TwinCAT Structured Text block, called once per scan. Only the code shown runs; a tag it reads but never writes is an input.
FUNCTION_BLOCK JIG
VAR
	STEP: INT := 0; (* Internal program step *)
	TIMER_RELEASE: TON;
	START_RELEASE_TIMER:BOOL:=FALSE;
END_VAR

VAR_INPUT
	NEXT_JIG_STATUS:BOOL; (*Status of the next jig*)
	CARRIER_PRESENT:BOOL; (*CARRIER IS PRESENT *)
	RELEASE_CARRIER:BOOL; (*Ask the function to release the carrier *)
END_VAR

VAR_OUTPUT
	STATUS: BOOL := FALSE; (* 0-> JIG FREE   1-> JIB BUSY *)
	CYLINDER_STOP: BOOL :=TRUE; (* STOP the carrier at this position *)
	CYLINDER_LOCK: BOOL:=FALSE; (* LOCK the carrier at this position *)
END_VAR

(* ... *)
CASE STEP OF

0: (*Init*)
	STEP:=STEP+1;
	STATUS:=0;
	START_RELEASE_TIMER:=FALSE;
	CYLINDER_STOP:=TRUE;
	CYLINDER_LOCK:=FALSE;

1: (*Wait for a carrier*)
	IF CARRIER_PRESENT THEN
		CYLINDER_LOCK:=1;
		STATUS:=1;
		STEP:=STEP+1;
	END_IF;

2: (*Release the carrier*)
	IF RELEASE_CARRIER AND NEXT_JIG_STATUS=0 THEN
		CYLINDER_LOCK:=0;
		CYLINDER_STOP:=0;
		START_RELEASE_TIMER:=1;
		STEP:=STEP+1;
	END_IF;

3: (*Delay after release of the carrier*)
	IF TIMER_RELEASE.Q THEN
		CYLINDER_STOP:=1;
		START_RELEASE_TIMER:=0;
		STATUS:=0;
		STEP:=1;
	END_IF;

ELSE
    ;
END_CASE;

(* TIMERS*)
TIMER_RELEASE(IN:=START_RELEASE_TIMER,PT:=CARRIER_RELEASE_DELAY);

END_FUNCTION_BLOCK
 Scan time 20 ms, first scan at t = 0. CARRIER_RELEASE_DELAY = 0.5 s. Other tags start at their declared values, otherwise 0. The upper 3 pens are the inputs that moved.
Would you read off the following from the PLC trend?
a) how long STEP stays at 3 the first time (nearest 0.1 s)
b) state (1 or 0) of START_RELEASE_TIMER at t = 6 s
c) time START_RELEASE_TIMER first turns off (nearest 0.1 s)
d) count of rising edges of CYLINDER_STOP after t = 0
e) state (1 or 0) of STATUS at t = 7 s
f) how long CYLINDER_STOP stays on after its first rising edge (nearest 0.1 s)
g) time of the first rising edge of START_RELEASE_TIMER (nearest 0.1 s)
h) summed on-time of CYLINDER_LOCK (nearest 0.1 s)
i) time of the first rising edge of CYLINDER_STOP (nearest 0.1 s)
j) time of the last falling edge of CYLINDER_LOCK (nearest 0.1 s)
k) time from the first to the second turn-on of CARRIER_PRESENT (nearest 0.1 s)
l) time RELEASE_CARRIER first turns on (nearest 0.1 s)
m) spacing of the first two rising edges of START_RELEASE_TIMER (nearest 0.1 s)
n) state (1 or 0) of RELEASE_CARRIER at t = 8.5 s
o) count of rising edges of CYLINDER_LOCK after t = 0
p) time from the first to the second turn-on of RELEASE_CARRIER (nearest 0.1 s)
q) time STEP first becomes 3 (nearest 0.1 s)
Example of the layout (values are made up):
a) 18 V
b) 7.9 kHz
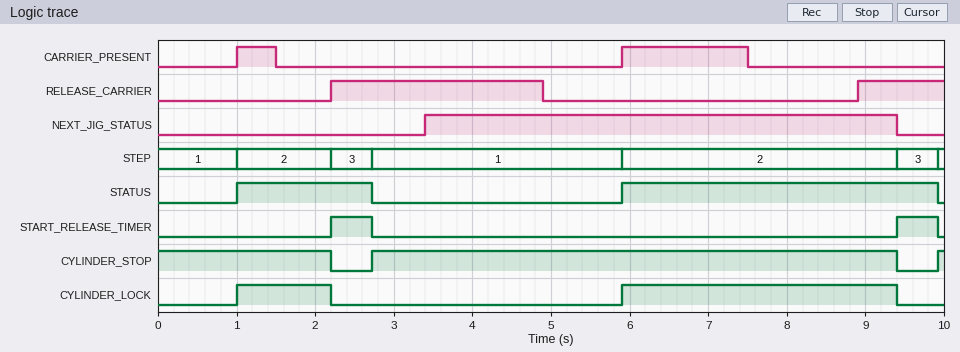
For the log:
a) 0.5 s
b) 0
c) 2.7 s
d) 2
e) 1
f) 6.7 s
g) 2.2 s
h) 4.7 s
i) 2.7 s
j) 9.4 s
k) 4.9 s
l) 2.2 s
m) 7.2 s
n) 0
o) 2
p) 6.7 s
q) 2.2 s
